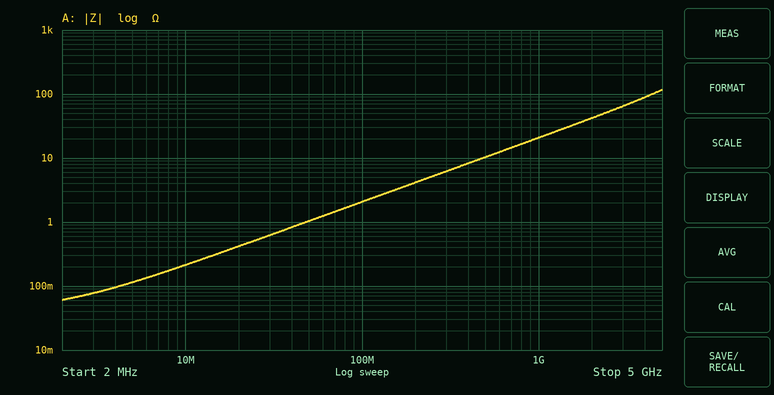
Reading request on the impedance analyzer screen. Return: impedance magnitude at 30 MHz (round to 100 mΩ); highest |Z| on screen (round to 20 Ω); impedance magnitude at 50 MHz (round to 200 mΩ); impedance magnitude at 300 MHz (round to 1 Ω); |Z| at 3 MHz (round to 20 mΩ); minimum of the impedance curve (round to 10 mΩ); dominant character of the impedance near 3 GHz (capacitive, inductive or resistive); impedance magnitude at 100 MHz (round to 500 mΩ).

600 mΩ
120 Ω
1.0 Ω
6 Ω
80 mΩ
60 mΩ
inductive
2.0 Ω
